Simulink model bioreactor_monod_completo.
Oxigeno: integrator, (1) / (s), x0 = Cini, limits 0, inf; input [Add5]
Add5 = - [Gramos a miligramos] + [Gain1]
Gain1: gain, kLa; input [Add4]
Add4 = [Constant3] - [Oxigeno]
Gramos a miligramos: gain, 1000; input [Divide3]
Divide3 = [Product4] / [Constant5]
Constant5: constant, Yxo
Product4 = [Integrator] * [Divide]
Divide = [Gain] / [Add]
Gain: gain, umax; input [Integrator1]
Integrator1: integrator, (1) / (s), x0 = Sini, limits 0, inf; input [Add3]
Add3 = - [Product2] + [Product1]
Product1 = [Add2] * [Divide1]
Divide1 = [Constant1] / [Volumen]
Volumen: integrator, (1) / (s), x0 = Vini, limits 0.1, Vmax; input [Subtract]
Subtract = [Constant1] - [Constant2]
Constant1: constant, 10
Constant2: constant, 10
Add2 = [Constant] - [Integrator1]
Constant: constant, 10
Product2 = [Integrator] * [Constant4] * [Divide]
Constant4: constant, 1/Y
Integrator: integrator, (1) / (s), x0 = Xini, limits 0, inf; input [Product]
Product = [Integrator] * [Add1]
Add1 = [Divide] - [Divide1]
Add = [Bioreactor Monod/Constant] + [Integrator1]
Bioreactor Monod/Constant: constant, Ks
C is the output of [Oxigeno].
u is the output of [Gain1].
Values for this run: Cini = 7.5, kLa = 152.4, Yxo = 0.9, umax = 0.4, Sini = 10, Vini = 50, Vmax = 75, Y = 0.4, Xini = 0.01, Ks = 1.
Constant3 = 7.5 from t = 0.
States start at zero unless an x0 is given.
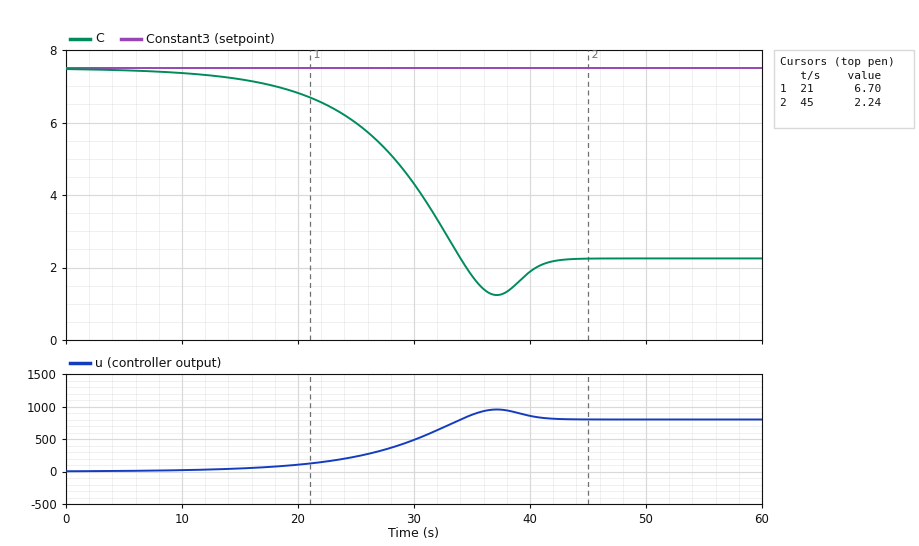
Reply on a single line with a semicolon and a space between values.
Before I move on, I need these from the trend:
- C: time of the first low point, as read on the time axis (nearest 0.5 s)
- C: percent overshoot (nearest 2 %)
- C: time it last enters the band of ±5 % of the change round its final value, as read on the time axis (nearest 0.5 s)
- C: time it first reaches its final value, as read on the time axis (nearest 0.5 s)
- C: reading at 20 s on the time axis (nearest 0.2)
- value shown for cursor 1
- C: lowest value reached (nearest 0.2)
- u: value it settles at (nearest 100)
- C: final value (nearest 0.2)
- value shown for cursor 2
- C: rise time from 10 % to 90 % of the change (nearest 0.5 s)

37.0 s; 20 %; 40.5 s; 34.0 s; 6.8; 6.70; 1.2; 800; 2.2; 2.24; 14.5 s
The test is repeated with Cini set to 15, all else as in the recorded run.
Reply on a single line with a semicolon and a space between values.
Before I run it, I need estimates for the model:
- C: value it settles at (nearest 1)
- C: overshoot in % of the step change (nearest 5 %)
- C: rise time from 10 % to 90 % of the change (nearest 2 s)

2; 10 %; 32 s
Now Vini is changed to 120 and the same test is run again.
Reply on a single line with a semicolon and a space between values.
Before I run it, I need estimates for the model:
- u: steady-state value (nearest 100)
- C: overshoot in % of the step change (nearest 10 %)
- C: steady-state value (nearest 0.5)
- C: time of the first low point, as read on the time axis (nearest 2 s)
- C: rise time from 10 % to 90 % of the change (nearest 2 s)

600; 70 %; 4.0; 26 s; 10 s
